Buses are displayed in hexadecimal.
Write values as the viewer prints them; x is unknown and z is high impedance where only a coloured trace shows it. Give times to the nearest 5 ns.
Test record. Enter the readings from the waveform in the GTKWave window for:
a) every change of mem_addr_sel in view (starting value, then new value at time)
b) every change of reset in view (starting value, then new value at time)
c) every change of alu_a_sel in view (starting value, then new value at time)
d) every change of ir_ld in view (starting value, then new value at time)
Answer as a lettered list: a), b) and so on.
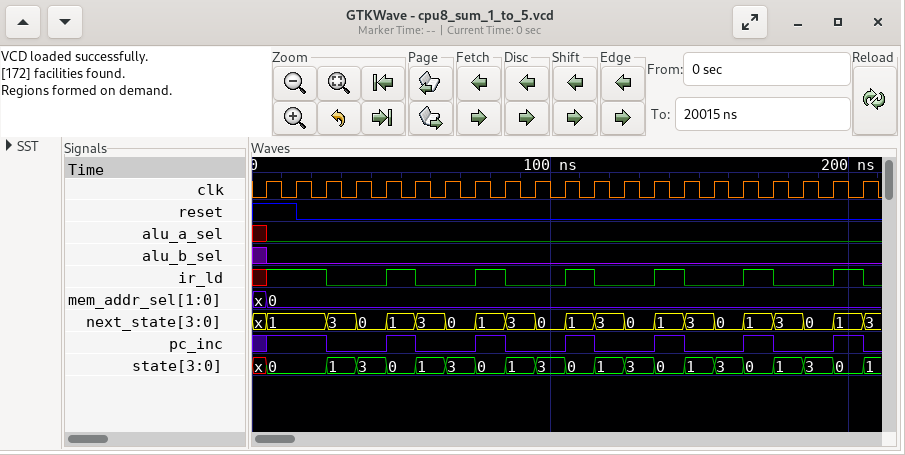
a) x, 0 at 5 ns
b) 1, 0 at 15 ns
c) x, 0 at 5 ns
d) x, 1 at 5 ns, 0 at 25 ns, 1 at 45 ns, 0 at 55 ns, 1 at 75 ns, 0 at 85 ns, 1 at 105 ns, 0 at 115 ns, 1 at 135 ns, 0 at 145 ns, 1 at 165 ns, 0 at 175 ns, 1 at 195 ns, 0 at 205 ns
